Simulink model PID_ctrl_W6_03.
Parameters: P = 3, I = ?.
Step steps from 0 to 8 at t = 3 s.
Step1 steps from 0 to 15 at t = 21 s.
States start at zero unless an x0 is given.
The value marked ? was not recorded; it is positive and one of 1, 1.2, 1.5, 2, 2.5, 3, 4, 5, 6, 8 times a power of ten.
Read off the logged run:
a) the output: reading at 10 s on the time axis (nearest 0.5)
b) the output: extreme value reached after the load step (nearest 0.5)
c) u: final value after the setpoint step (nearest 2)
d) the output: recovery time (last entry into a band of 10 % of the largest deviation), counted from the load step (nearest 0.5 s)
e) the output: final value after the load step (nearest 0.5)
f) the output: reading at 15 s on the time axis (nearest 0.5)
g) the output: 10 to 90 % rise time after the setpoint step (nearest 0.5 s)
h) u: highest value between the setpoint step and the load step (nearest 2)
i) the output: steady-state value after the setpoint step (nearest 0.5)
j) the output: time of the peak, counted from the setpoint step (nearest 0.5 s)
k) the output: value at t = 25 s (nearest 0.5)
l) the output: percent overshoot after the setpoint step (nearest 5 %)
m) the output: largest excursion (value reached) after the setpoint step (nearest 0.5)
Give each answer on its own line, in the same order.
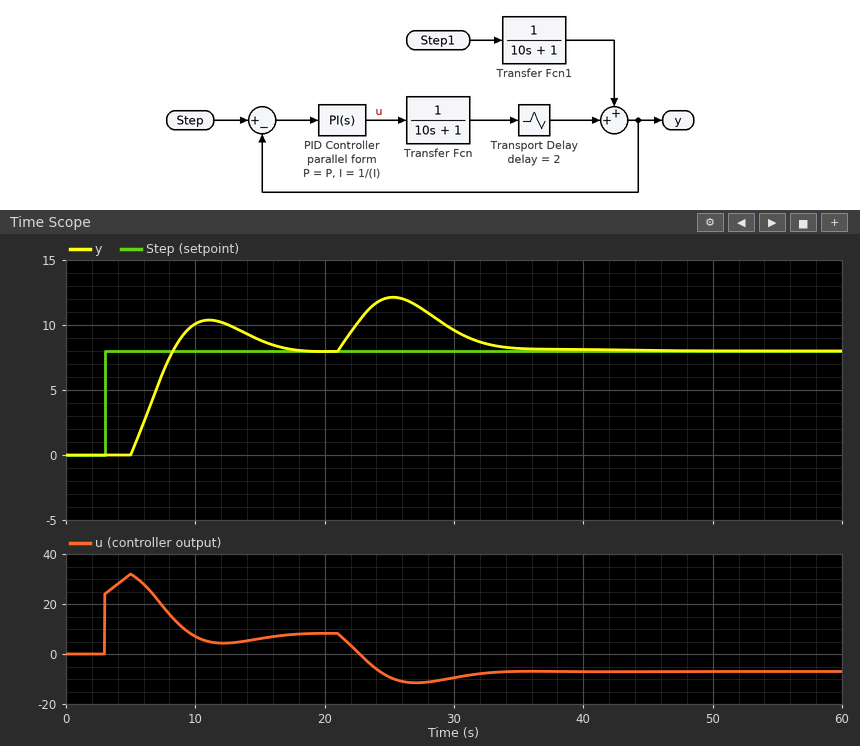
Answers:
10.0
12.0
8
12.0 s
8.0
9.0
2.5 s
32
8.0
8.0 s
12.0
30 %
10.5
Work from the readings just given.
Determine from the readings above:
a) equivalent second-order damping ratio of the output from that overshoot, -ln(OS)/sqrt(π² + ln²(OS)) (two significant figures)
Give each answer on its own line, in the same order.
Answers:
0.36
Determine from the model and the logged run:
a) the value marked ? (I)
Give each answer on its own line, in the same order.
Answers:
2
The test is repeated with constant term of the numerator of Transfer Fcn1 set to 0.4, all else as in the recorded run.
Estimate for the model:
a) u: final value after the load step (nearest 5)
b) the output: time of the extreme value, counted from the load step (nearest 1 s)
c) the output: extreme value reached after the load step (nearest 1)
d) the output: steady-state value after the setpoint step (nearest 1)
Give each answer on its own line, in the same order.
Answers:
0
4 s
10
8
